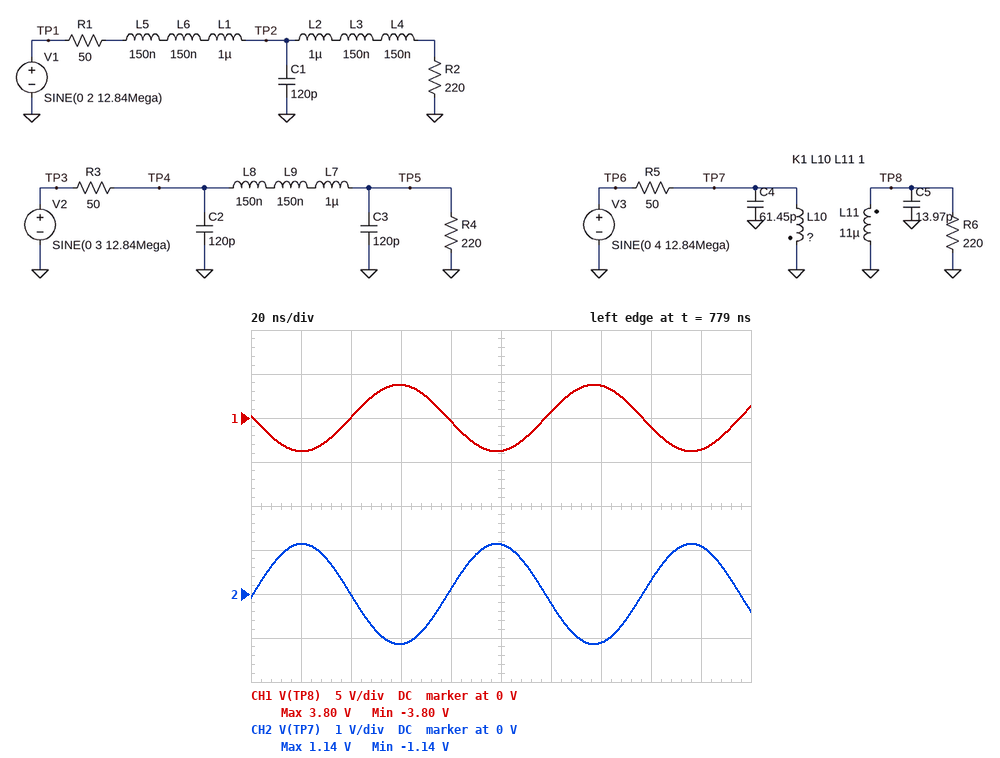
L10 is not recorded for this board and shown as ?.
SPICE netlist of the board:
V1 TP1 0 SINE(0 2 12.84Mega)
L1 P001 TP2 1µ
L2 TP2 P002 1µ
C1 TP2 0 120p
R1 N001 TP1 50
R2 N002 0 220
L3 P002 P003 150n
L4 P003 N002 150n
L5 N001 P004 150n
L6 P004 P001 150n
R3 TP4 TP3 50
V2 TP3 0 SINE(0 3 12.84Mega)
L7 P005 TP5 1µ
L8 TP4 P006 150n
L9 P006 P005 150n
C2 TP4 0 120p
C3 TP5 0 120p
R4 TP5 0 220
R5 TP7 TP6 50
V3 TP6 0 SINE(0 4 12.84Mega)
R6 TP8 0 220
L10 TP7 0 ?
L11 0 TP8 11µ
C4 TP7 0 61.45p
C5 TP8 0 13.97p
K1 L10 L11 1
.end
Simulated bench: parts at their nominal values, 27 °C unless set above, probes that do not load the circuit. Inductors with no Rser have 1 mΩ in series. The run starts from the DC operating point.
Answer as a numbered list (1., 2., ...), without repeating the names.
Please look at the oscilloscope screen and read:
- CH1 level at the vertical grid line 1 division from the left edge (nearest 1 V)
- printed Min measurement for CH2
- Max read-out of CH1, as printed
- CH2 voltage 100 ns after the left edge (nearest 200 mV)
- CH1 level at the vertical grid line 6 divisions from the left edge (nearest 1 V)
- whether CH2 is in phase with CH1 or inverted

1. -4 V
2. -1.14 V
3. 3.80 V
4. 1.2 V
5. 1 V
6. inverted
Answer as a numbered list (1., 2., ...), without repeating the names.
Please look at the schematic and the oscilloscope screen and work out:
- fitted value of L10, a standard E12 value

1. 1 µH
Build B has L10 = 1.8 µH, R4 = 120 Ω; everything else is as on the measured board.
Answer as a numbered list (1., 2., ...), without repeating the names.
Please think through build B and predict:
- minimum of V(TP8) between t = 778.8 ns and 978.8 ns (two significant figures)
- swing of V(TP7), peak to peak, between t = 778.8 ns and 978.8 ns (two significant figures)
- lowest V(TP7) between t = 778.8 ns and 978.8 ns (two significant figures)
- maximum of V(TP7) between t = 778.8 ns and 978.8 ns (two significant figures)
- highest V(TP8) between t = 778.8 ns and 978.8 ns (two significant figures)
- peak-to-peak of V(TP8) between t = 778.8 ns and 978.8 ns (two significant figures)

1. -4.1 V
2. 3.3 V
3. -1.7 V
4. 1.7 V
5. 4.1 V
6. 8.2 V
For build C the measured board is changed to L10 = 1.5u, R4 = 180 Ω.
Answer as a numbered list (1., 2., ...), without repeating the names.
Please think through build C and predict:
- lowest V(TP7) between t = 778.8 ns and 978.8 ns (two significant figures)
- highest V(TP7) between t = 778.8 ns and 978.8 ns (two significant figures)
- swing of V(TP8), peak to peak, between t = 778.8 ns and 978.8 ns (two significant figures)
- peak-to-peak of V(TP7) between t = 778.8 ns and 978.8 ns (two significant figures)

1. -1.5 V
2. 1.5 V
3. 8.1 V
4. 3.0 V
